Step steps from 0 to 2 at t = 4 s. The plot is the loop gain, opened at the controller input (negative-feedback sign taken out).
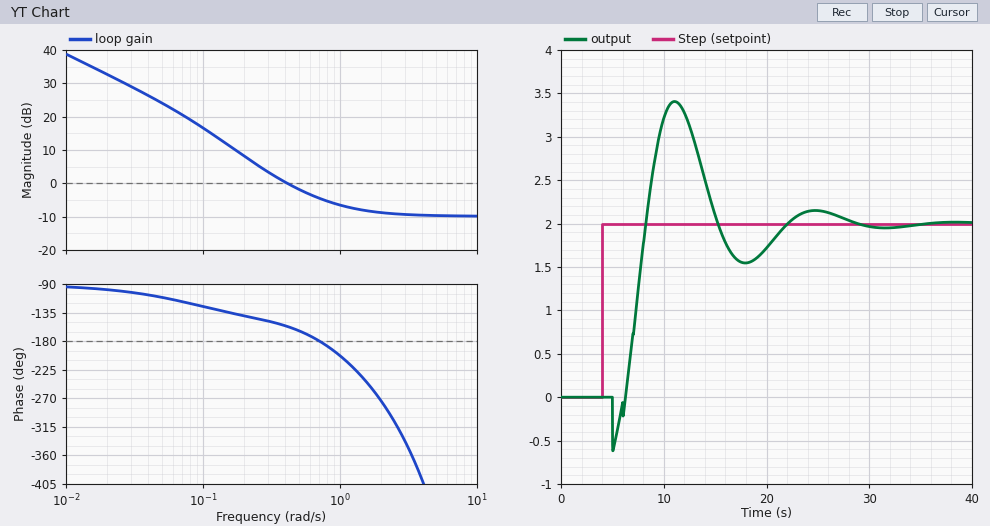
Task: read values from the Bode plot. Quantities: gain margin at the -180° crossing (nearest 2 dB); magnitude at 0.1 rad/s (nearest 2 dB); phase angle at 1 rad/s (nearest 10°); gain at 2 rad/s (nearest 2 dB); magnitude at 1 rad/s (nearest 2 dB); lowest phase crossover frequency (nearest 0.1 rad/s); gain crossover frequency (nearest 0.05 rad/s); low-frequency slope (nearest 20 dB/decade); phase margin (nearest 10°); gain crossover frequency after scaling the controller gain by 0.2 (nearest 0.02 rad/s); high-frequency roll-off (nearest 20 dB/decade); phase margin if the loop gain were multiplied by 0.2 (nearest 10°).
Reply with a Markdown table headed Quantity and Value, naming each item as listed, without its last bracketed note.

| Quantity | Value |
|---|---|
| gain margin at the -180° crossing | 4 dB |
| magnitude at 0.1 rad/s | 16 dB |
| phase angle at 1 rad/s | -200° |
| gain at 2 rad/s | -8 dB |
| magnitude at 1 rad/s | -6 dB |
| lowest phase crossover frequency | 0.7 rad/s |
| gain crossover frequency | 0.40 rad/s |
| low-frequency slope | -20 dB/decade |
| phase margin | 20° |
| gain crossover frequency after scaling the controller gain by 0.2 | 0.12 rad/s |
| high-frequency roll-off | 0 dB/decade |
| phase margin if the loop gain were multiplied by 0.2 | 50° |
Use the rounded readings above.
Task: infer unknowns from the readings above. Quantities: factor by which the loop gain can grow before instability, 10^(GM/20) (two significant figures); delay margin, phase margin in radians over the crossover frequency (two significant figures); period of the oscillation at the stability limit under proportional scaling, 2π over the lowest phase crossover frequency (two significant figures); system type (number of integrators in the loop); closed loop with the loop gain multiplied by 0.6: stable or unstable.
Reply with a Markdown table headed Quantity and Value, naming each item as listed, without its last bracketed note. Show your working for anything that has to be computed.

| Quantity | Value |
|---|---|
| factor by which the loop gain can grow before instability, 10^(GM/20) | 10^(4 / 20) = 1.6 |
| delay margin, phase margin in radians over the crossover frequency | 20 × π / 180 / 0.4 = 0.87 s |
| period of the oscillation at the stability limit under proportional scaling, 2π over the lowest phase crossover frequency | 2π / 0.7 = 9.0 s |
| system type | 1 |
| closed loop with the loop gain multiplied by 0.6: stable or unstable | stable |
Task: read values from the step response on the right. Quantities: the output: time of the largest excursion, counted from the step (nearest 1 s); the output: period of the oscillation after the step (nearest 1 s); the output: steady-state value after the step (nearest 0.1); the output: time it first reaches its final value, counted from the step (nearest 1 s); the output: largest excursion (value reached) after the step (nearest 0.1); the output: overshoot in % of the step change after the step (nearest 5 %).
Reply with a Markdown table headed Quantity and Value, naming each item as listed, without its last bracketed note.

| Quantity | Value |
|---|---|
| the output: time of the largest excursion, counted from the step | 7 s |
| the output: period of the oscillation after the step | 14 s |
| the output: steady-state value after the step | 2.0 |
| the output: time it first reaches its final value, counted from the step | 4 s |
| the output: largest excursion (value reached) after the step | 3.4 |
| the output: overshoot in % of the step change after the step | 70 % |
